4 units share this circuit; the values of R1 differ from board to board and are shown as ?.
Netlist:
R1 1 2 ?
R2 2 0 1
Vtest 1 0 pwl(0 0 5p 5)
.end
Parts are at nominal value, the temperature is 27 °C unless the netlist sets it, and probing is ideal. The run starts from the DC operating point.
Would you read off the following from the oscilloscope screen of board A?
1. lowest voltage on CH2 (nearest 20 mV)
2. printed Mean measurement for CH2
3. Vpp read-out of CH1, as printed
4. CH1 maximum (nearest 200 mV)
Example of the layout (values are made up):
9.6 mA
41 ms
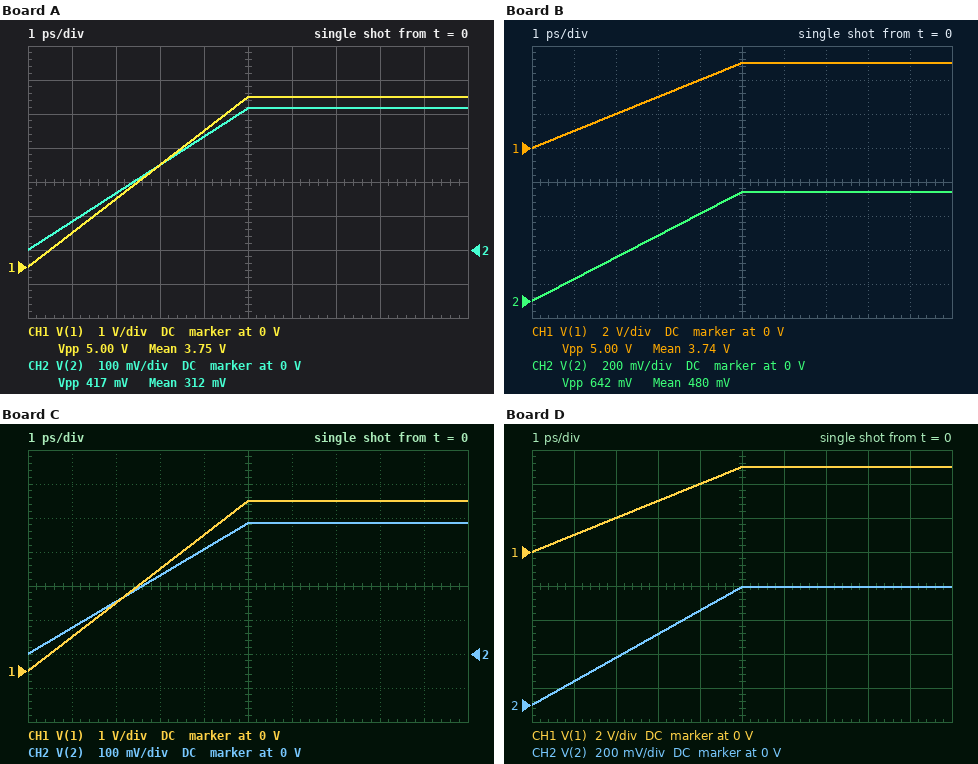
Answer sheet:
0 V
312 mV
5.00 V
5.0 V
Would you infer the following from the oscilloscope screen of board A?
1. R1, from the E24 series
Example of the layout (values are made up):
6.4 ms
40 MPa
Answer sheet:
11 Ω
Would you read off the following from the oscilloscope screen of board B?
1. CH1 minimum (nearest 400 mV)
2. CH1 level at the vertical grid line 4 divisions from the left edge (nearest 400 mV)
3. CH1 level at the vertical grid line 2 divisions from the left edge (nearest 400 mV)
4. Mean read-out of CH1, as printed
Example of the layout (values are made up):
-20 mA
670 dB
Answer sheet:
0 V
4.0 V
2.0 V
3.74 V
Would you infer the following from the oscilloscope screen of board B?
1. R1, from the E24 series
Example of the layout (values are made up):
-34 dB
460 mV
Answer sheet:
6.8 Ω
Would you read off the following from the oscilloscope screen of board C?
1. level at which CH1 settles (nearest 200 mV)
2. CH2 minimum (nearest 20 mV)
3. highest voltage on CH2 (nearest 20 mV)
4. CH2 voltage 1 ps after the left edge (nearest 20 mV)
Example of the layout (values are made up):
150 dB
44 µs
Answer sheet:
5.0 V
0 V
380 mV
80 mV
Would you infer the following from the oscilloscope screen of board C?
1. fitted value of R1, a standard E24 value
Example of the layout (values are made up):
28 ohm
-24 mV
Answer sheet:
12 Ω
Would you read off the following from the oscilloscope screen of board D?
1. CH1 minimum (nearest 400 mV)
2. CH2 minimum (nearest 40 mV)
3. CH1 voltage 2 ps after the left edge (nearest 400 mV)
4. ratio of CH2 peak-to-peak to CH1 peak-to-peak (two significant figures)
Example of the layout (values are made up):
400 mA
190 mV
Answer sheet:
0 V
0 V
2.0 V
0.14
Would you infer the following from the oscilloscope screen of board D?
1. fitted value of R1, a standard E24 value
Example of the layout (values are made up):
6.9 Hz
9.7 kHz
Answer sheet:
6.2 Ω
